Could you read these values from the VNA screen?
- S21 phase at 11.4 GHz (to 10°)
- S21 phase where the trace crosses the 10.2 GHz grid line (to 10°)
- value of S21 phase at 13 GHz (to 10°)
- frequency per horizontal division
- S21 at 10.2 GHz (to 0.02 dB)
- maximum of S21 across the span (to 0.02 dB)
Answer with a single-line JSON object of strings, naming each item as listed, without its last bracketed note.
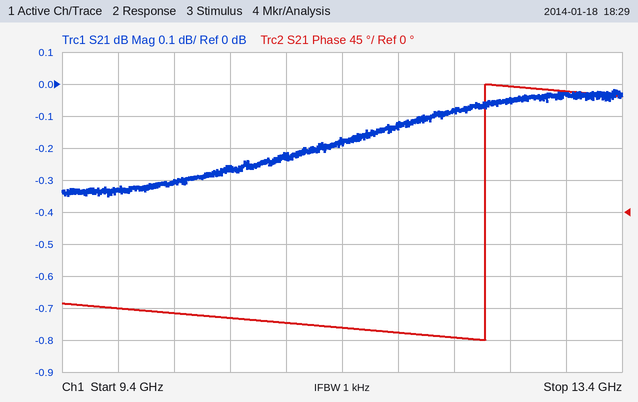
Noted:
{"S21 phase at 11.4 GHz": "-160°", "S21 phase where the trace crosses the 10.2 GHz grid line": "-140°", "value of S21 phase at 13 GHz": "170°", "frequency per horizontal division": "400 MHz", "S21 at 10.2 GHz": "-0.30 dB", "maximum of S21 across the span": "-0.02 dB"}
